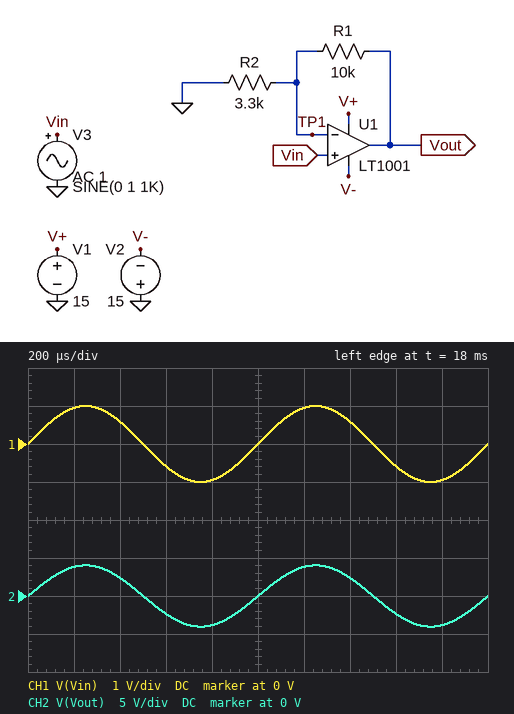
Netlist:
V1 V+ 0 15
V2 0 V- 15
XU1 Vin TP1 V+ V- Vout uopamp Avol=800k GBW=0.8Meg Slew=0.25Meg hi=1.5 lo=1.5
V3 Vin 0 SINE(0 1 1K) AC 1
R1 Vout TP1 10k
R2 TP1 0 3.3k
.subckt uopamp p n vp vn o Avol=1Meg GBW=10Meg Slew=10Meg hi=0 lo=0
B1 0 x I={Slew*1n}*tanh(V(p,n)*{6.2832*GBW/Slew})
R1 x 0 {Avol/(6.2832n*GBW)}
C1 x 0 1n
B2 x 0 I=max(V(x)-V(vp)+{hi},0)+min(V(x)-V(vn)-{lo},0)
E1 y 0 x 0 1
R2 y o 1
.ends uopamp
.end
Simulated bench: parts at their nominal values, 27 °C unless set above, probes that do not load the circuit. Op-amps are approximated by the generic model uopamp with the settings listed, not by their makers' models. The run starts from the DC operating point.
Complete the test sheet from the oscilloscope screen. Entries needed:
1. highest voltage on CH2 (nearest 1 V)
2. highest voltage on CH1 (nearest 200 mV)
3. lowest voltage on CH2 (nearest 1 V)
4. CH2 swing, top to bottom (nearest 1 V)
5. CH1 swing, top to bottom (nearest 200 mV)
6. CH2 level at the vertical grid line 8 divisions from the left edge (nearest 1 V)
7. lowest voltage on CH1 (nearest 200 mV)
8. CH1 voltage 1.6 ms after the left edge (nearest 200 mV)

4 V
1.0 V
-4 V
8 V
2.0 V
-2 V
-1.0 V
-600 mV
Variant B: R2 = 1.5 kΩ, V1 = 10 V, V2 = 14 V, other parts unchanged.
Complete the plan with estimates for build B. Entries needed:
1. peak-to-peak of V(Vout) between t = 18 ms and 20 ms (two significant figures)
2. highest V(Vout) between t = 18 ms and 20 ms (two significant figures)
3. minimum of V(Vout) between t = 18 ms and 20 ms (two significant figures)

15 V
7.7 V
-7.7 V
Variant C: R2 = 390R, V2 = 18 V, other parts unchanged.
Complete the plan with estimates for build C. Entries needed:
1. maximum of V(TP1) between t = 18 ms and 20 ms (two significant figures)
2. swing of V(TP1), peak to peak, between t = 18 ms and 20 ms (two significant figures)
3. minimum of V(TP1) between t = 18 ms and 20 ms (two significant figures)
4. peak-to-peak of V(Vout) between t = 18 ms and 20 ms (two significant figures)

510 mV
1.1 V
-620 mV
30 V
